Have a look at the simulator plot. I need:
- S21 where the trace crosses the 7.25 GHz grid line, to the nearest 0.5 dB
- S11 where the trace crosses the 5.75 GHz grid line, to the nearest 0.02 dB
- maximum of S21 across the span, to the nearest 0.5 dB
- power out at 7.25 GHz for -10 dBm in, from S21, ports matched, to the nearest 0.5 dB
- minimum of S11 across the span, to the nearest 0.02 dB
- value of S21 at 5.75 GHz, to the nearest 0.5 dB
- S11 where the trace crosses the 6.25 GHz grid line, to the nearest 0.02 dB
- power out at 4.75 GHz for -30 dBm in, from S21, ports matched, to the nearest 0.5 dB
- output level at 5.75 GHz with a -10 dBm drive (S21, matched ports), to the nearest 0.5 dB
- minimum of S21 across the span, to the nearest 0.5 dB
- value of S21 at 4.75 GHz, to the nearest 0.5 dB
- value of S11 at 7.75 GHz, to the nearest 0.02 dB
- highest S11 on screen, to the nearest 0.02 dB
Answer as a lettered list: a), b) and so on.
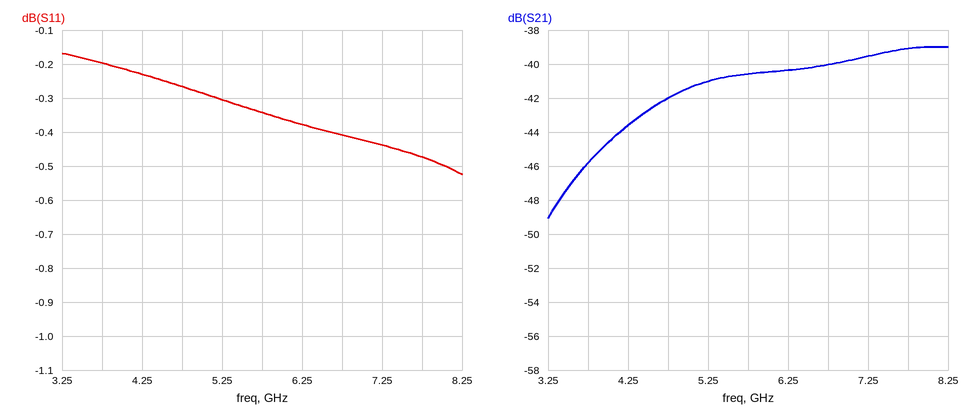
a) -39.5 dB
b) -0.34 dB
c) -39.0 dB
d) -49.5 dBm
e) -0.52 dB
f) -40.5 dB
g) -0.38 dB
h) -72.0 dBm
i) -50.5 dBm
j) -49.0 dB
k) -42.0 dB
l) -0.48 dB
m) -0.16 dB
